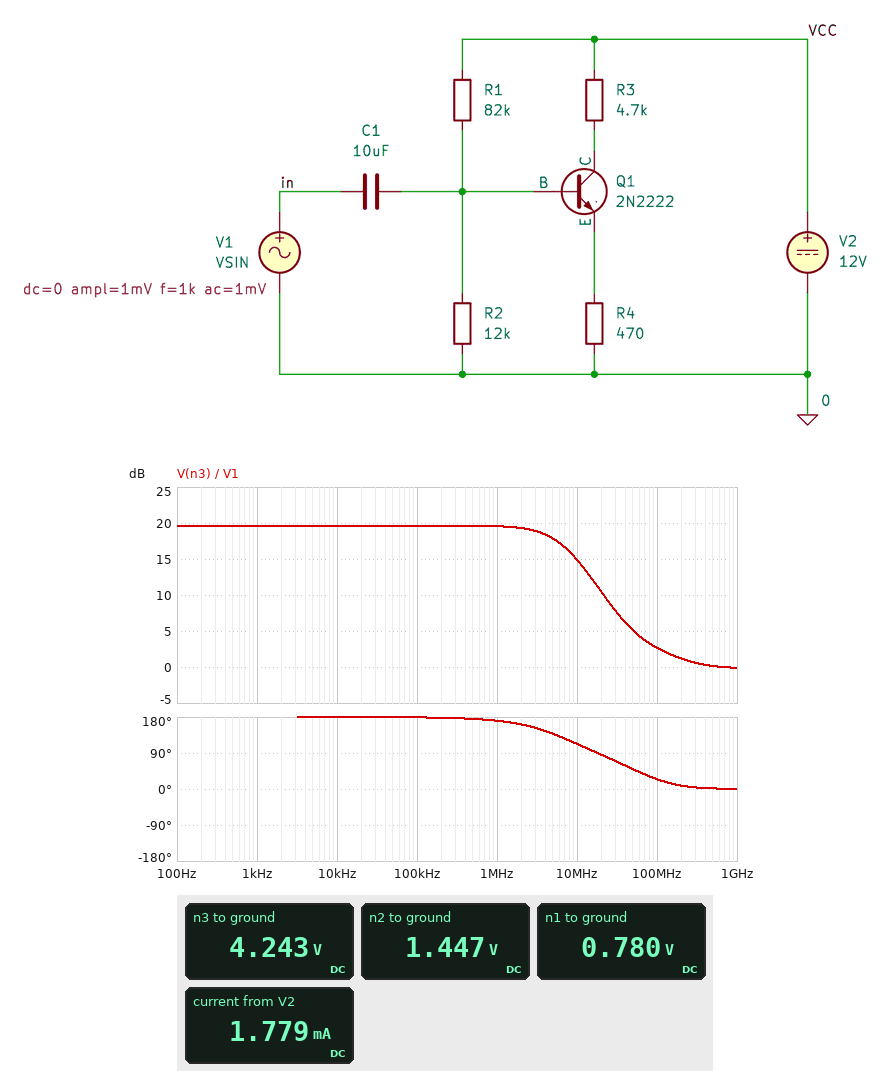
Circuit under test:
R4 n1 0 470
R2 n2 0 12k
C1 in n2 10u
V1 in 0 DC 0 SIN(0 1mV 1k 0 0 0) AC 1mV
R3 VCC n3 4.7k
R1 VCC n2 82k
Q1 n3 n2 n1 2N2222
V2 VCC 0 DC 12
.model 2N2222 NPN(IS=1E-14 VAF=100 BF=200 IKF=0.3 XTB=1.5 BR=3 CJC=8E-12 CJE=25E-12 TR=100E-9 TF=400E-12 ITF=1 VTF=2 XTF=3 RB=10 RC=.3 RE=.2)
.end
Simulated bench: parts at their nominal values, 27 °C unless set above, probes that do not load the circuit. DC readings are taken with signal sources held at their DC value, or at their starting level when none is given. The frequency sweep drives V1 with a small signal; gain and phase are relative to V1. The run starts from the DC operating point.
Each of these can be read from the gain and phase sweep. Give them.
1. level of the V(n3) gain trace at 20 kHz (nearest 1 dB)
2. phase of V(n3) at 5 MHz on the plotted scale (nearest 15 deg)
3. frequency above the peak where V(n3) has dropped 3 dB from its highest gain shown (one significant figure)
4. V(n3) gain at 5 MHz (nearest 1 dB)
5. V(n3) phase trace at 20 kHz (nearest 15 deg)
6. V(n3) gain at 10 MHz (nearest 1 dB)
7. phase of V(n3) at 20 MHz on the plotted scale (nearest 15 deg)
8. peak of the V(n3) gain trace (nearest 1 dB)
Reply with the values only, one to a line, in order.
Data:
20 dB
135 deg
7 MHz
18 dB
180 deg
15 dB
90 deg
20 dB
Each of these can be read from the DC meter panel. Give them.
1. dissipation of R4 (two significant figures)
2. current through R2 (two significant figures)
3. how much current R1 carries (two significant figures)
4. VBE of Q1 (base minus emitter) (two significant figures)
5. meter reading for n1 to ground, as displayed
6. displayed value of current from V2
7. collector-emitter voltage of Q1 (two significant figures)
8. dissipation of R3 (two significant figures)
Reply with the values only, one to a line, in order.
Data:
1.3 mW
120 µA
130 µA
670 mV
0.780 V
1.779 mA
3.5 V
13 mW
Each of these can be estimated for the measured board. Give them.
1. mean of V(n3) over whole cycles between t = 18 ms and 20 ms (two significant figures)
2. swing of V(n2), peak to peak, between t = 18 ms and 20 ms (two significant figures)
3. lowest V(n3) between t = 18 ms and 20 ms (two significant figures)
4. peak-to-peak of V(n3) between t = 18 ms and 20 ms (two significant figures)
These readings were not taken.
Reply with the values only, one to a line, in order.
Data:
4.2 V
2.0 mV
4.2 V
19 mV
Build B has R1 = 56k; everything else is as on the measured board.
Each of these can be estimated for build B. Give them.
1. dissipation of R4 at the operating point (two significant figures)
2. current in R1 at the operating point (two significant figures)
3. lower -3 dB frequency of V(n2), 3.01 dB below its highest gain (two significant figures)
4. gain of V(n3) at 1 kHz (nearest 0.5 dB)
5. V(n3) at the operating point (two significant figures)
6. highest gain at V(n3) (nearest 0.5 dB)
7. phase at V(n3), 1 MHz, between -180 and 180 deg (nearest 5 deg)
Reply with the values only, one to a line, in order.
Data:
2.6 mW
180 µA
29 Hz
-0.5 dB
1.2 V
0 dB
65 deg
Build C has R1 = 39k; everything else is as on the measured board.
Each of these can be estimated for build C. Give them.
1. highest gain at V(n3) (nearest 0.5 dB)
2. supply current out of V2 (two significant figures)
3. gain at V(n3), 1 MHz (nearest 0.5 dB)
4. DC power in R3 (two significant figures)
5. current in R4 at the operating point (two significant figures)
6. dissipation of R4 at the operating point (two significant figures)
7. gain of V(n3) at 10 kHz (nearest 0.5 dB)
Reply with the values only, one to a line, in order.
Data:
0 dB
2.6 mA
-1.0 dB
25 mW
2.4 mA
2.7 mW
-7.0 dB
